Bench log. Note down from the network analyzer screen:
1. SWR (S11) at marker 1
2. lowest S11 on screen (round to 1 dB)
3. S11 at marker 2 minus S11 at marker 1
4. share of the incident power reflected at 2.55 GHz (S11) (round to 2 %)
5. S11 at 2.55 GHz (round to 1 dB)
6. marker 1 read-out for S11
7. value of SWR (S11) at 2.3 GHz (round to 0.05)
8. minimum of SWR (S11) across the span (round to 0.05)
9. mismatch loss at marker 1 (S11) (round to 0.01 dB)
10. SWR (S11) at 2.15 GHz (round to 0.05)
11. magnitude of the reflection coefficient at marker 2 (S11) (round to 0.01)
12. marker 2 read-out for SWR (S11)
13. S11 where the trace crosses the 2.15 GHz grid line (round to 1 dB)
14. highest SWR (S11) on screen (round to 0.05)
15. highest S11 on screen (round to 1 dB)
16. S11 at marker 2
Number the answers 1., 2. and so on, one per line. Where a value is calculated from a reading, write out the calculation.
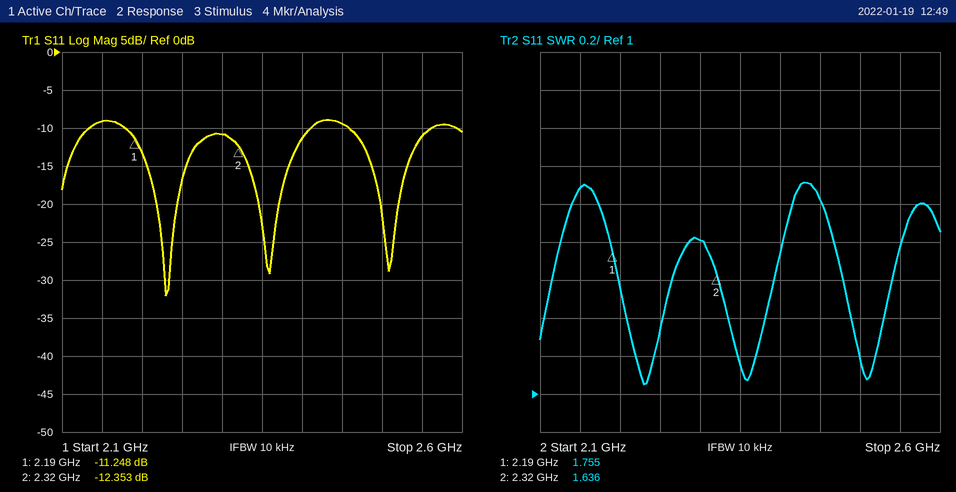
1. 1.755
2. -32 dB
3. -12.353 − (-11.248) = -1.105 dB
4. 10^(-11/10) ≈ 8 %
5. -11 dB
6. -11.248 dB
7. 1.80
8. 1.05
9. −10 log10(1 − 10^(-11.248/10)) ≈ 0.34 dB
10. 2.10
11. 10^(-12.353/20) ≈ 0.24
12. 1.636
13. -9 dB
14. 2.10
15. -9 dB
16. -12.353 dB
